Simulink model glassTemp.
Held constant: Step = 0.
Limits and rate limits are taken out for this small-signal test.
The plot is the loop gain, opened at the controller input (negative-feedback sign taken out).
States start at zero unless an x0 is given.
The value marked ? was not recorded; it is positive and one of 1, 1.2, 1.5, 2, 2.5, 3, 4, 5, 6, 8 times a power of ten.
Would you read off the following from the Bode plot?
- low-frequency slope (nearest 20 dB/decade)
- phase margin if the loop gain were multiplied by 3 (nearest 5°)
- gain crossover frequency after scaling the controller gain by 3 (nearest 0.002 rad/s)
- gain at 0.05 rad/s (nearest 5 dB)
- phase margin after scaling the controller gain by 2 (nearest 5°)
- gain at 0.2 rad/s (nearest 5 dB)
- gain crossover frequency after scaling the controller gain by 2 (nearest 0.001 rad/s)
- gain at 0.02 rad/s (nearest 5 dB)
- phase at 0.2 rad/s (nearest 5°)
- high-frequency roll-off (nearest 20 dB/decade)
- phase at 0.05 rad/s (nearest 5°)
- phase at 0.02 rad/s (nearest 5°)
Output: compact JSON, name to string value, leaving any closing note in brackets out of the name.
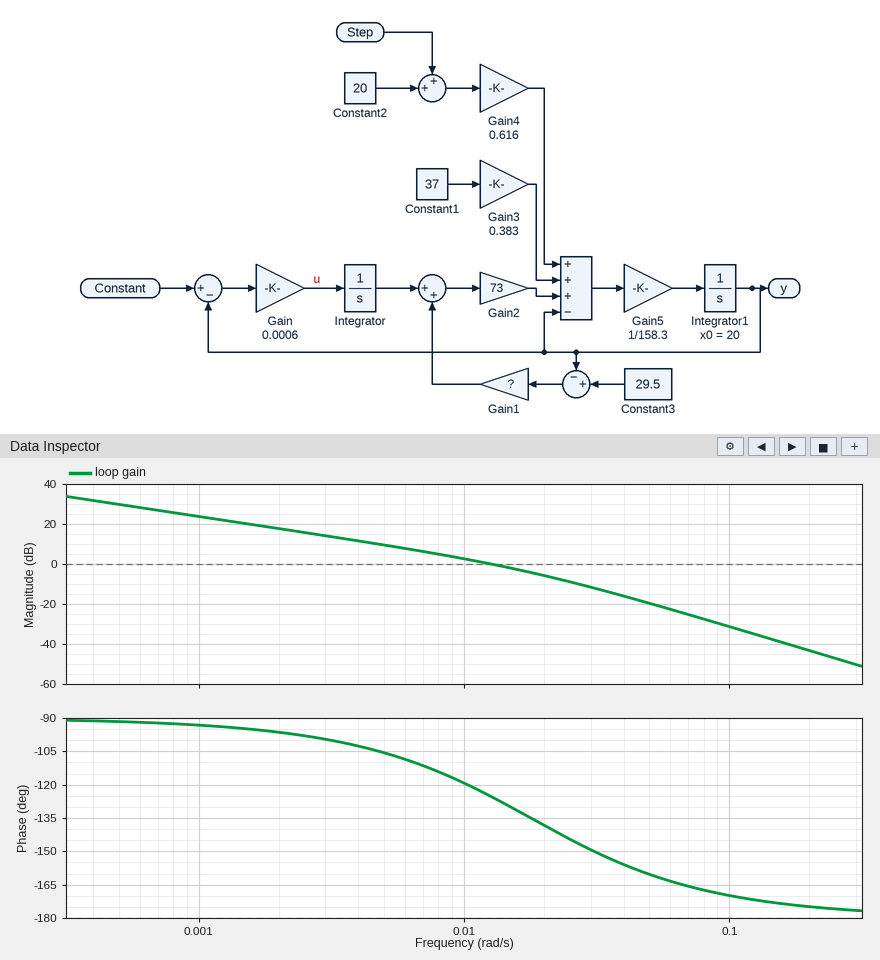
{"low-frequency slope": "-20 dB/decade", "phase margin if the loop gain were multiplied by 3": "35°", "gain crossover frequency after scaling the controller gain by 3": "0.026 rad/s", "gain at 0.05 rad/s": "-20 dB", "phase margin after scaling the controller gain by 2": "40°", "gain at 0.2 rad/s": "-45 dB", "gain crossover frequency after scaling the controller gain by 2": "0.020 rad/s", "gain at 0.02 rad/s": "-5 dB", "phase at 0.2 rad/s": "-175°", "high-frequency roll-off": "-40 dB/decade", "phase at 0.05 rad/s": "-160°", "phase at 0.02 rad/s": "-140°"}
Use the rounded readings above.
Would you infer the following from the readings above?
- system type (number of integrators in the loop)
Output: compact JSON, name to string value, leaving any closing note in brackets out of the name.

{"system type": "1"}
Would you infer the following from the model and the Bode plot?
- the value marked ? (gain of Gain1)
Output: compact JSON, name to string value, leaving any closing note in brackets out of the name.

{"the value marked ?": "0.025"}
